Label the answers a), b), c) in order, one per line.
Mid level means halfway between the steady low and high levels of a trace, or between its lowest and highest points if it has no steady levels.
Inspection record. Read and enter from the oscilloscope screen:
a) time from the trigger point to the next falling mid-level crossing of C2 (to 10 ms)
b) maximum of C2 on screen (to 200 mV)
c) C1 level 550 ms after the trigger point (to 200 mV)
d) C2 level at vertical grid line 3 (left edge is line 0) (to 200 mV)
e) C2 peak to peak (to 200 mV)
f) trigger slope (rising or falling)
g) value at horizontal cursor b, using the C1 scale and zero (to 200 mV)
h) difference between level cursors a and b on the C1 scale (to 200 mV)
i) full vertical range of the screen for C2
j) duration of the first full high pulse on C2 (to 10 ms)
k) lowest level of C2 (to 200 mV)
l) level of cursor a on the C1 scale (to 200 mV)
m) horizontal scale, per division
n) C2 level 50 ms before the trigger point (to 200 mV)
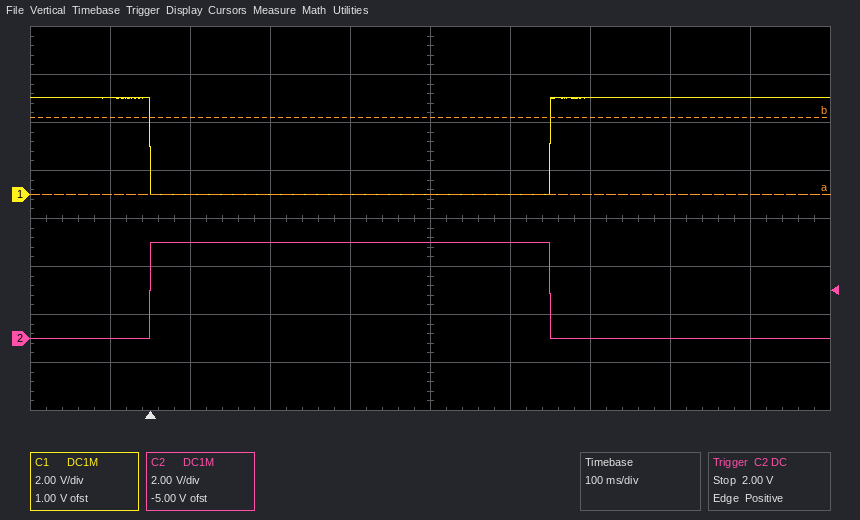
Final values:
a) 500 ms
b) 4.0 V
c) 4.0 V
d) 4.0 V
e) 4.0 V
f) rising
g) 3.2 V
h) 3.2 V
i) 16 V
j) 500 ms
k) 0.0 V
l) 0.0 V
m) 100 ms
n) 0.0 V
